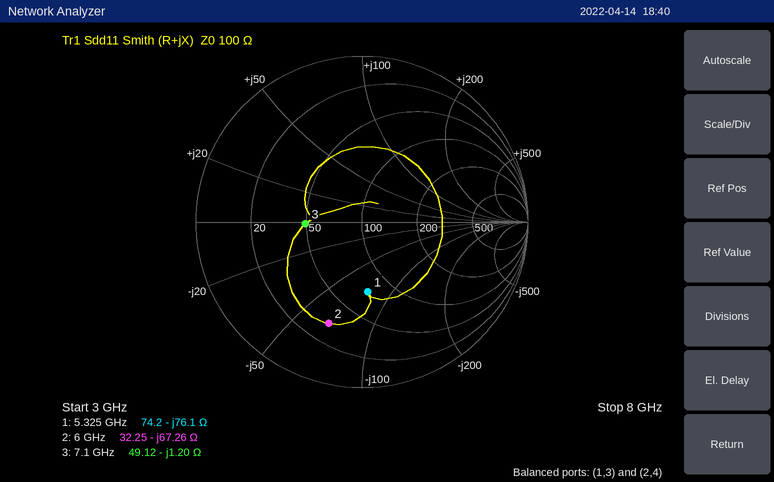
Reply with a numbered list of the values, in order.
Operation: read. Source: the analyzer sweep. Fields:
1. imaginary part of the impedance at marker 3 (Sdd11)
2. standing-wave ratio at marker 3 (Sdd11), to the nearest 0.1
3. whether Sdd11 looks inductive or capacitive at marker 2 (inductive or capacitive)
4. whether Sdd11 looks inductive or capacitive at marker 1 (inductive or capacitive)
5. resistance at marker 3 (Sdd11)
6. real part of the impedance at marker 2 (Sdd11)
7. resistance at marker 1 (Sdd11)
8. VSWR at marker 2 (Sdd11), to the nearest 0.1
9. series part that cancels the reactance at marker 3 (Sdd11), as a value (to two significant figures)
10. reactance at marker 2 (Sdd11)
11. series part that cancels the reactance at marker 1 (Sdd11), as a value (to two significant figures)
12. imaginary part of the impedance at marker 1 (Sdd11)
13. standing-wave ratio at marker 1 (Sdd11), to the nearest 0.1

1. -1.20 Ω
2. 2.0
3. capacitive
4. capacitive
5. 49.12 Ω
6. 32.25 Ω
7. 74.2 Ω
8. 4.6
9. 27 pH
10. -67.26 Ω
11. 2.3 nH
12. -76.1 Ω
13. 2.5
